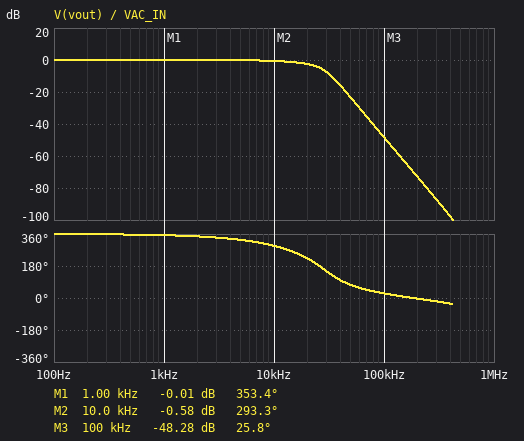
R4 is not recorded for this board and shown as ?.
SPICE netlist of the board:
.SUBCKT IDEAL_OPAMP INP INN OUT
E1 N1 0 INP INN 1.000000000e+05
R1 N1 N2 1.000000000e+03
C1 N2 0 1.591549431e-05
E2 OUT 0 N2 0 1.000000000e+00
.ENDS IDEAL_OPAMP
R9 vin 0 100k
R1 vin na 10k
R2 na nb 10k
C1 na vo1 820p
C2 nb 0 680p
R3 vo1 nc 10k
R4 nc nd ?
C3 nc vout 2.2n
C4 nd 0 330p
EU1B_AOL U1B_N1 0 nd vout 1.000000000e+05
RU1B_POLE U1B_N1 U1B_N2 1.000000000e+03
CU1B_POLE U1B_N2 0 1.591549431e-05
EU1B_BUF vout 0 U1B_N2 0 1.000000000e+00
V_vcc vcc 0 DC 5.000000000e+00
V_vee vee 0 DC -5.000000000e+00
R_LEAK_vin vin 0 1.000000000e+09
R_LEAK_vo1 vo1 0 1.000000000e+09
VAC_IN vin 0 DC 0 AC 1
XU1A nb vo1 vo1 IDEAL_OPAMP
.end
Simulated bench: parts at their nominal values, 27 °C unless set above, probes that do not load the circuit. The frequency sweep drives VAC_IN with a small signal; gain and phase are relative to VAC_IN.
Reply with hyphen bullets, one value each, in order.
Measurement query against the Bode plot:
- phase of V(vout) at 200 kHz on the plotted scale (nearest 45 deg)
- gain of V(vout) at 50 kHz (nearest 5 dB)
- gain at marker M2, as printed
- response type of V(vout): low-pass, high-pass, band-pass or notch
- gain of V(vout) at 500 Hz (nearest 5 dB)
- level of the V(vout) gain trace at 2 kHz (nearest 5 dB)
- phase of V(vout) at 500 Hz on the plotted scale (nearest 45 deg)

- 0 deg
- -25 dB
- -0.58 dB
- low-pass
- 0 dB
- 0 dB
- 360 deg
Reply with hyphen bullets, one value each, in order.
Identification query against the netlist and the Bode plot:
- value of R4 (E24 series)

- 3.6 kΩ
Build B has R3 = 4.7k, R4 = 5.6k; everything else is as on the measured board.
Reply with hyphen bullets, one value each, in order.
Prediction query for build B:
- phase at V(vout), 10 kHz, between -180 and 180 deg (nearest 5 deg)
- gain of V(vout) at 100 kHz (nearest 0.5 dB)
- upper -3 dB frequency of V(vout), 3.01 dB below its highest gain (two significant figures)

- -60 deg
- -45.0 dB
- 21 kHz
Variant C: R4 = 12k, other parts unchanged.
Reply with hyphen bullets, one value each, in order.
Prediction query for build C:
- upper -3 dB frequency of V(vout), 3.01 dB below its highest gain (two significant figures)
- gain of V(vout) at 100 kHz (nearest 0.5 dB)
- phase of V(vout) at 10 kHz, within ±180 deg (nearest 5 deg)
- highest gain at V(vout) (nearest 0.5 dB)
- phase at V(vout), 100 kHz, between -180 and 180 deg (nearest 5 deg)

- 18 kHz
- -58.5 dB
- -85 deg
- 1.0 dB
- 20 deg
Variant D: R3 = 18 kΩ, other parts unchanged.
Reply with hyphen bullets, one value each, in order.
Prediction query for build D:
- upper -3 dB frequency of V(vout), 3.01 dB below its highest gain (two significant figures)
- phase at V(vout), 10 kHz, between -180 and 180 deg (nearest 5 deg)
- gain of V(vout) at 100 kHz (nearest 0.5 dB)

- 19 kHz
- -80 deg
- -53.5 dB
